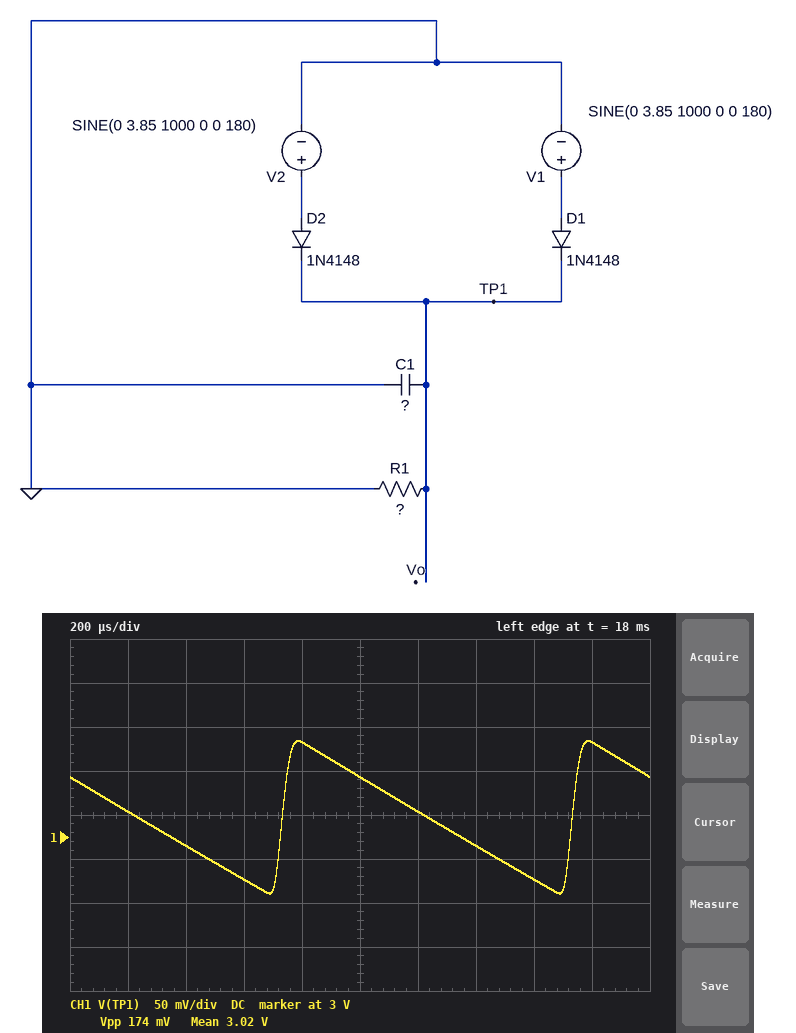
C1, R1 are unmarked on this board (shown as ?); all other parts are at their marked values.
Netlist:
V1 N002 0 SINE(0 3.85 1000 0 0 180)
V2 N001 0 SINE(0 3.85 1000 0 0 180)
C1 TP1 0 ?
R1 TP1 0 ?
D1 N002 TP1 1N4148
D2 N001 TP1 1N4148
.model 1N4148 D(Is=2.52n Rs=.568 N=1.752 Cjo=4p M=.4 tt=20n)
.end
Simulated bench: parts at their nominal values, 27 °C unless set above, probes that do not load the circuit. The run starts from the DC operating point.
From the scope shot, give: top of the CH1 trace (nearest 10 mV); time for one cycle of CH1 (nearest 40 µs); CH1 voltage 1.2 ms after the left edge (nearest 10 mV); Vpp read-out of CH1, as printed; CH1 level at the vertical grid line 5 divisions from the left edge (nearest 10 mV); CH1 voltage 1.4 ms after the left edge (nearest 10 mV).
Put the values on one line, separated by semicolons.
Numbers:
3.11 V; 1.00 ms; 3.03 V; 174 mV; 3.07 V; 2.99 V
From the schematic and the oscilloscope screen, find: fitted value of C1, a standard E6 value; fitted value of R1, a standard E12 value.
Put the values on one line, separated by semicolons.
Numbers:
33 µF; 470 Ω
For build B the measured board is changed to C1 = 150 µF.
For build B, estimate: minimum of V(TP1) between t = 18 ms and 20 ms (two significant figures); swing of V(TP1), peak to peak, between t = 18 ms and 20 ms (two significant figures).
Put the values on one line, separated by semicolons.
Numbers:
3.0 V; 39 mV
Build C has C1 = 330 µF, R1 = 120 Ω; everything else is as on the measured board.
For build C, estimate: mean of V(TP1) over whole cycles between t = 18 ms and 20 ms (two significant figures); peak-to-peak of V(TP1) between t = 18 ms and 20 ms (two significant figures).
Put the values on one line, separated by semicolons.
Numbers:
2.9 V; 65 mV
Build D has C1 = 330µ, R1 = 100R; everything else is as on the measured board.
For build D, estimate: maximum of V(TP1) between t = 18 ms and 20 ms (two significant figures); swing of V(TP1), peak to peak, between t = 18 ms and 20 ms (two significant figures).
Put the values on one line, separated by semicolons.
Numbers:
2.9 V; 77 mV
